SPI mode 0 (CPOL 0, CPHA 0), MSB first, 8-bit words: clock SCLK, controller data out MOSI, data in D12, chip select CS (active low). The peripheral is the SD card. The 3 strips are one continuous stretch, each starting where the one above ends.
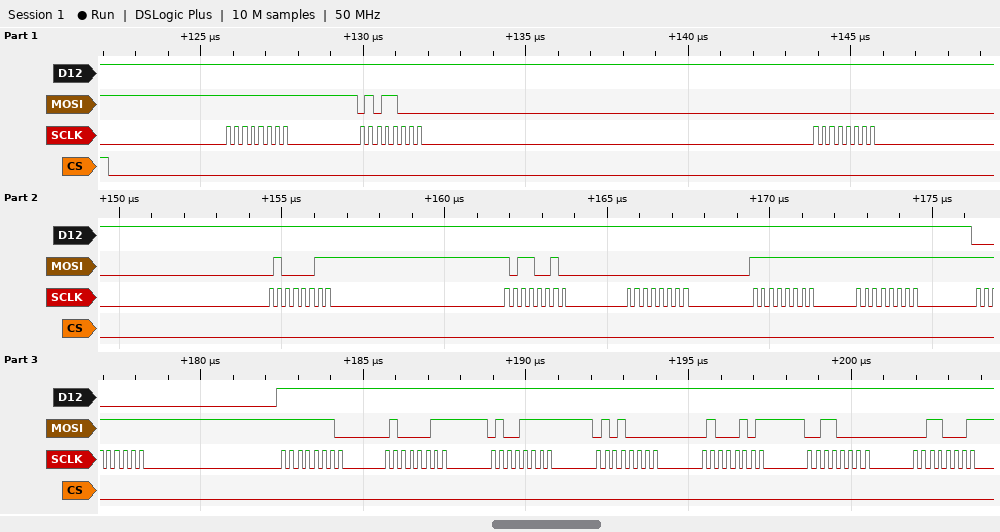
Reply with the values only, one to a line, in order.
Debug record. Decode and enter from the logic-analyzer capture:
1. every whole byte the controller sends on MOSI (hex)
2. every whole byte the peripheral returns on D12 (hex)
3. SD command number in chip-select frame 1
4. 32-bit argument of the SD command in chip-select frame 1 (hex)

FF 58 00 43 B2 00 FF FF FF FE 43 4F 50 45 30 31
FF FF FF FF FF FF FF FF 00 FF FF FF FF FF FF FF
CMD24
0x0043B200
